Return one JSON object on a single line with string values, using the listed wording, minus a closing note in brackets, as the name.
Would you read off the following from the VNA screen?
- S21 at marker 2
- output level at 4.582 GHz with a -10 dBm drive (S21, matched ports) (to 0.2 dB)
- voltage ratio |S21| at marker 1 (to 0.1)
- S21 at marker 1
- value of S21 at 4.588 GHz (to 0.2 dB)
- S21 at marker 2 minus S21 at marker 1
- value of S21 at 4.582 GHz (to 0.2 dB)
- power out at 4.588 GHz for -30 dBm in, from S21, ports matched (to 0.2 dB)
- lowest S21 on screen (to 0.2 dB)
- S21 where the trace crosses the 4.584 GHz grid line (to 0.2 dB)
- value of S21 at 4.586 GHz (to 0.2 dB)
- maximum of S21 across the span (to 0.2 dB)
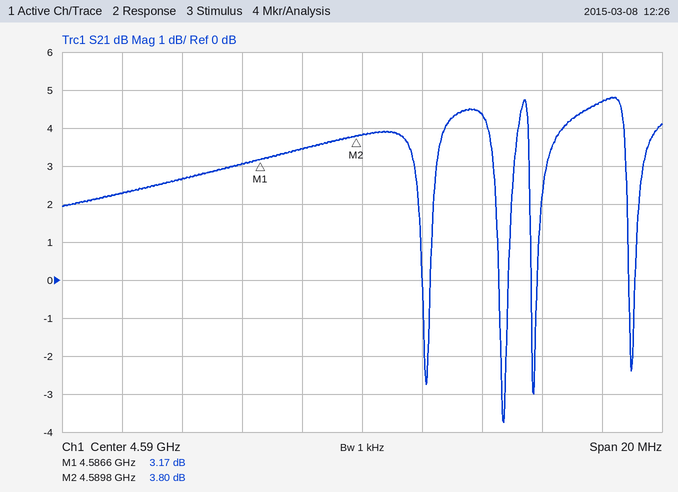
{"S21 at marker 2": "3.80 dB", "output level at 4.582 GHz with a -10 dBm drive (S21, matched ports)": "-7.8 dBm", "voltage ratio |S21| at marker 1": "1.4", "S21 at marker 1": "3.17 dB", "value of S21 at 4.588 GHz": "3.4 dB", "S21 at marker 2 minus S21 at marker 1": "0.63 dB", "value of S21 at 4.582 GHz": "2.2 dB", "power out at 4.588 GHz for -30 dBm in, from S21, ports matched": "-26.6 dBm", "lowest S21 on screen": "-3.8 dB", "S21 where the trace crosses the 4.584 GHz grid line": "2.6 dB", "value of S21 at 4.586 GHz": "3.0 dB", "maximum of S21 across the span": "4.8 dB"}
